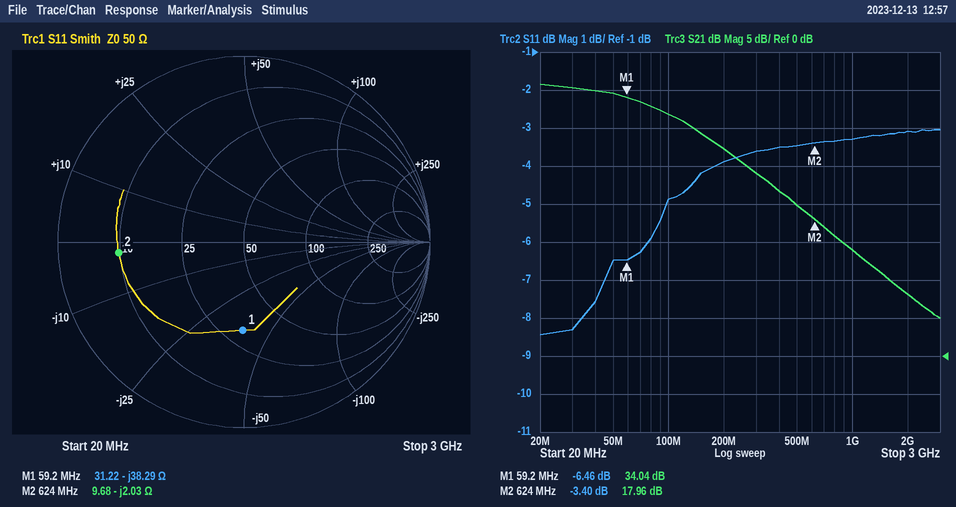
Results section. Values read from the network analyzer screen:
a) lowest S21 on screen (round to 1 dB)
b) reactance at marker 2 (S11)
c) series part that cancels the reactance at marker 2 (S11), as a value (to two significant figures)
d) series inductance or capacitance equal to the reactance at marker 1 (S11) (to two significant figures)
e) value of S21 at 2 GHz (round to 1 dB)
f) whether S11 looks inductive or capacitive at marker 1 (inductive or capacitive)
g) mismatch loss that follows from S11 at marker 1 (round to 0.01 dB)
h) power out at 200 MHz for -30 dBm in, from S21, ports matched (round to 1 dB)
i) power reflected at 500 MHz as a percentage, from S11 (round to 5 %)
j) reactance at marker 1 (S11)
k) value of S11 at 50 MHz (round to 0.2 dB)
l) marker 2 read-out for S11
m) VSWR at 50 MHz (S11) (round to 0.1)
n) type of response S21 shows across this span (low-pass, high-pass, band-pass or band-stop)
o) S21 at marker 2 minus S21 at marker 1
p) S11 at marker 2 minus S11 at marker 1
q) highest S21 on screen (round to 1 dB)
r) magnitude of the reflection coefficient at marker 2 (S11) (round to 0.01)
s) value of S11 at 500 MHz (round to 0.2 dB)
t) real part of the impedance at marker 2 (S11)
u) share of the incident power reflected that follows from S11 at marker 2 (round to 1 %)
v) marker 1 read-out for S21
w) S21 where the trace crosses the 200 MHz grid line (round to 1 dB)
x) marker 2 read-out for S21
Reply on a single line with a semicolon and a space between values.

5 dB; -2.03 Ω; 520 pH; 70 pF; 8 dB; capacitive; 1.11 dB; -3 dBm; 45 %; -38.29 Ω; -6.4 dB; -3.40 dB; 2.8; low-pass; -16.08 dB; 3.06 dB; 36 dB; 0.68; -3.4 dB; 9.68 Ω; 46 %; 34.04 dB; 27 dB; 17.96 dB
